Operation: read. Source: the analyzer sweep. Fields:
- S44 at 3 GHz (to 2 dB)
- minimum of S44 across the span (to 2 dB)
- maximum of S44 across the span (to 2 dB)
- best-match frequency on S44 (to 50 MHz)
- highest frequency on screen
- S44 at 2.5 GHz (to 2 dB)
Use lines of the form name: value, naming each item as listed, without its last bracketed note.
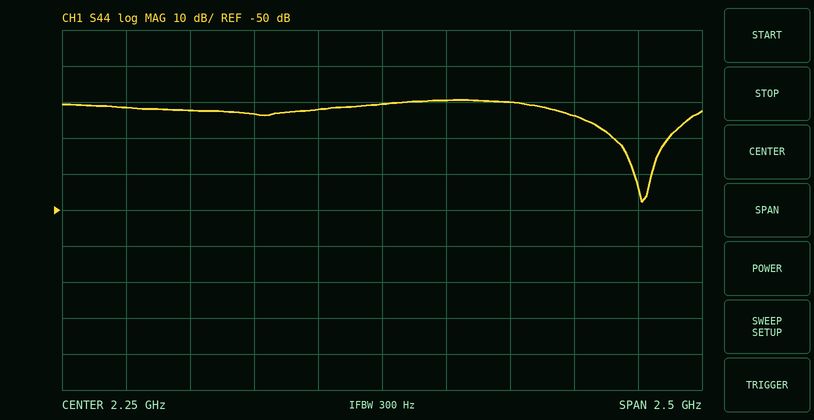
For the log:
S44 at 3 GHz: -24 dB
minimum of S44 across the span: -48 dB
maximum of S44 across the span: -20 dB
best-match frequency on S44: 3.25 GHz
highest frequency on screen: 3.5 GHz
S44 at 2.5 GHz: -20 dB
